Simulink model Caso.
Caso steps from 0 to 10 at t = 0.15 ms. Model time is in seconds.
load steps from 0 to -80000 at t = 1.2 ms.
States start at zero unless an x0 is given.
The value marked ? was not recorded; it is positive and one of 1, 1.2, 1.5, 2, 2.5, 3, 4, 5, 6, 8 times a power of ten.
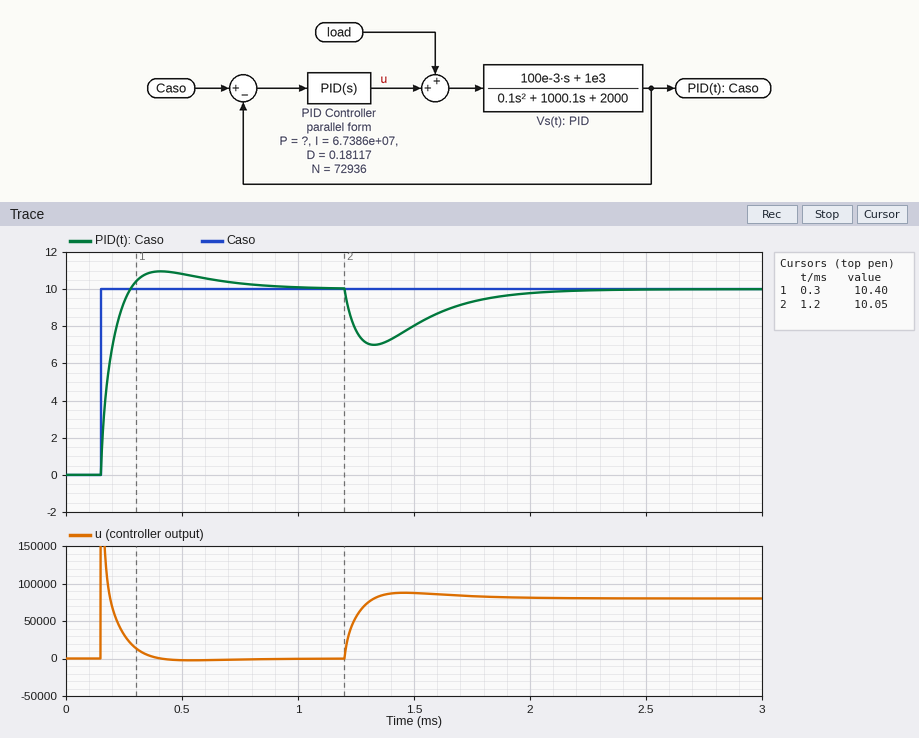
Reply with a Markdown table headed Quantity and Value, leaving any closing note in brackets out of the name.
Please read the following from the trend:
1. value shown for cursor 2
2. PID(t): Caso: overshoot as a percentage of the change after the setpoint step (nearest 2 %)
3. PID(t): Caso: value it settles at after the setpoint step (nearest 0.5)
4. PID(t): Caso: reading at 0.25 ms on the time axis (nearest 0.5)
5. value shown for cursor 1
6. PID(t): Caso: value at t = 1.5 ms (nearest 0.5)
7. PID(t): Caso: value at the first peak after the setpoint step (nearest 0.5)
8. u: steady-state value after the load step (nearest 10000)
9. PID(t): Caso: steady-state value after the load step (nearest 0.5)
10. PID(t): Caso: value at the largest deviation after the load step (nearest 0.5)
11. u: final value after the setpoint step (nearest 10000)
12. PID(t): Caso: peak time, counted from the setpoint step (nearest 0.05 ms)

| Quantity | Value |
|---|---|
| value shown for cursor 2 | 10.05 |
| PID(t): Caso: overshoot as a percentage of the change after the setpoint step | 10 % |
| PID(t): Caso: value it settles at after the setpoint step | 10.0 |
| PID(t): Caso: reading at 0.25 ms on the time axis | 9.5 |
| value shown for cursor 1 | 10.40 |
| PID(t): Caso: value at t = 1.5 ms | 8.0 |
| PID(t): Caso: value at the first peak after the setpoint step | 11.0 |
| u: steady-state value after the load step | 80000 |
| PID(t): Caso: steady-state value after the load step | 10.0 |
| PID(t): Caso: value at the largest deviation after the load step | 7.0 |
| u: final value after the setpoint step | 0 |
| PID(t): Caso: peak time, counted from the setpoint step | 0.25 ms |
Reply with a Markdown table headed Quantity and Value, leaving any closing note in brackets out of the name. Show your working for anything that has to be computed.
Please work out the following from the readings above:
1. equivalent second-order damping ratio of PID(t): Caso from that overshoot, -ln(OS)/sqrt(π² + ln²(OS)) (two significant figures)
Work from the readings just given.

| Quantity | Value |
|---|---|
| equivalent second-order damping ratio of PID(t): Caso from that overshoot, -ln(OS)/sqrt(π² + ln²(OS)) | ln(0.1) = -2.303; 2.303 / sqrt(9.870 + 5.302) = 0.59 |
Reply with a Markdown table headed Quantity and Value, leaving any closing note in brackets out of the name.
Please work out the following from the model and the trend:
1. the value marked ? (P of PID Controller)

| Quantity | Value |
|---|---|
| the value marked ? | 20000 |
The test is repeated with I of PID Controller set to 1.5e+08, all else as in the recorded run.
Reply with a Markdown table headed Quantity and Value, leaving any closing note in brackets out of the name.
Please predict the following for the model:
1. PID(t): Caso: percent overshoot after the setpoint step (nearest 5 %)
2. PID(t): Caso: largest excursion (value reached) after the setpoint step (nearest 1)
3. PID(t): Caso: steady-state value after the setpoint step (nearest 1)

| Quantity | Value |
|---|---|
| PID(t): Caso: percent overshoot after the setpoint step | 15 % |
| PID(t): Caso: largest excursion (value reached) after the setpoint step | 12 |
| PID(t): Caso: steady-state value after the setpoint step | 10 |
